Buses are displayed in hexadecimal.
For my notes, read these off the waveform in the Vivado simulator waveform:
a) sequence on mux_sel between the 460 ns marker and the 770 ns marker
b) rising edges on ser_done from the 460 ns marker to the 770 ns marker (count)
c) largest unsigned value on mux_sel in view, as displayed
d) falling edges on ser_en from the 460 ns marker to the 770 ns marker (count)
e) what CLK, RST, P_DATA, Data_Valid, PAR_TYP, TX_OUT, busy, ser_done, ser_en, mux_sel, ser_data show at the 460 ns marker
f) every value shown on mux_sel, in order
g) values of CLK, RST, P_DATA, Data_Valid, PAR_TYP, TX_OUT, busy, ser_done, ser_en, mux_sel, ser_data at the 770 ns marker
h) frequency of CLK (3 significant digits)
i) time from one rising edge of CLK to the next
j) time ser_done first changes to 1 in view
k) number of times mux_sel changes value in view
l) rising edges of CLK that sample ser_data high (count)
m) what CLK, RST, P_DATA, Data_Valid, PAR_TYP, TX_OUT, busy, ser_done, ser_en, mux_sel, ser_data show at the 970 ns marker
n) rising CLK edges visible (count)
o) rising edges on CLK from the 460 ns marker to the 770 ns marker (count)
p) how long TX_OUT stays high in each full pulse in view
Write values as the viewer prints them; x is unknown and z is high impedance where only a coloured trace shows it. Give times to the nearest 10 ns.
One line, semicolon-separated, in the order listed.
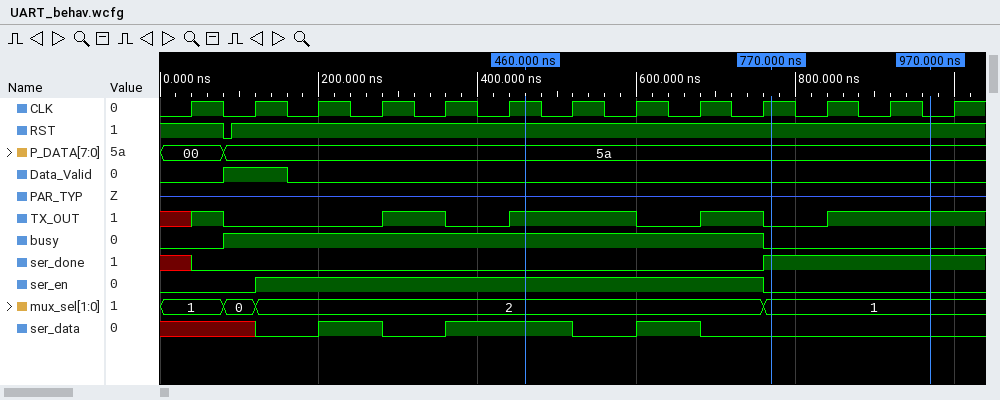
2, 1; 1; 2; 1; CLK=1, RST=1, P_DATA=5a, Data_Valid=0, PAR_TYP=z, TX_OUT=1, busy=1, ser_done=0, ser_en=1, mux_sel=2, ser_data=1; 1, 0, 2, 1; CLK=1, RST=1, P_DATA=5a, Data_Valid=0, PAR_TYP=z, TX_OUT=0, busy=0, ser_done=1, ser_en=0, mux_sel=1, ser_data=0; 12.5 MHz; 80 ns; 760 ns; 3; 4; CLK=0, RST=1, P_DATA=5a, Data_Valid=0, PAR_TYP=z, TX_OUT=1, busy=0, ser_done=1, ser_en=0, mux_sel=1, ser_data=0; 13; 4; 80 ns, 160 ns, 80 ns
